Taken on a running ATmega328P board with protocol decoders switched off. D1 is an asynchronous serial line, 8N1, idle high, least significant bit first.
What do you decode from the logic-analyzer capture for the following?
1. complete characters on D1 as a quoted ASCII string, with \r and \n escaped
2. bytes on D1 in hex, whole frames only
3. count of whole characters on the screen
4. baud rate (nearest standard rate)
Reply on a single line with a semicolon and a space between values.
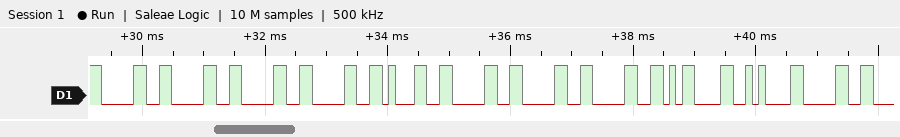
"00001000\r\n0"; 30 30 30 30 31 30 30 30 0D 0A 30; 11; 9600 baud
